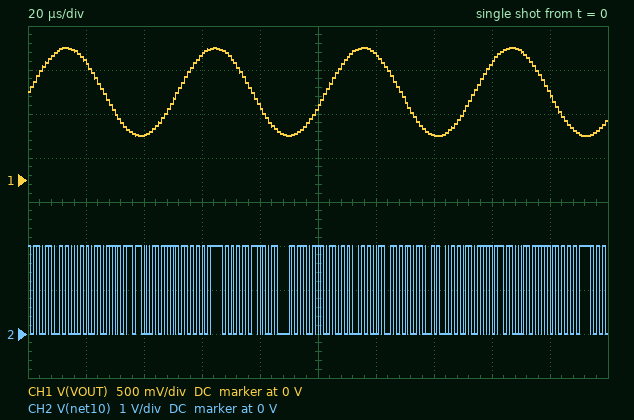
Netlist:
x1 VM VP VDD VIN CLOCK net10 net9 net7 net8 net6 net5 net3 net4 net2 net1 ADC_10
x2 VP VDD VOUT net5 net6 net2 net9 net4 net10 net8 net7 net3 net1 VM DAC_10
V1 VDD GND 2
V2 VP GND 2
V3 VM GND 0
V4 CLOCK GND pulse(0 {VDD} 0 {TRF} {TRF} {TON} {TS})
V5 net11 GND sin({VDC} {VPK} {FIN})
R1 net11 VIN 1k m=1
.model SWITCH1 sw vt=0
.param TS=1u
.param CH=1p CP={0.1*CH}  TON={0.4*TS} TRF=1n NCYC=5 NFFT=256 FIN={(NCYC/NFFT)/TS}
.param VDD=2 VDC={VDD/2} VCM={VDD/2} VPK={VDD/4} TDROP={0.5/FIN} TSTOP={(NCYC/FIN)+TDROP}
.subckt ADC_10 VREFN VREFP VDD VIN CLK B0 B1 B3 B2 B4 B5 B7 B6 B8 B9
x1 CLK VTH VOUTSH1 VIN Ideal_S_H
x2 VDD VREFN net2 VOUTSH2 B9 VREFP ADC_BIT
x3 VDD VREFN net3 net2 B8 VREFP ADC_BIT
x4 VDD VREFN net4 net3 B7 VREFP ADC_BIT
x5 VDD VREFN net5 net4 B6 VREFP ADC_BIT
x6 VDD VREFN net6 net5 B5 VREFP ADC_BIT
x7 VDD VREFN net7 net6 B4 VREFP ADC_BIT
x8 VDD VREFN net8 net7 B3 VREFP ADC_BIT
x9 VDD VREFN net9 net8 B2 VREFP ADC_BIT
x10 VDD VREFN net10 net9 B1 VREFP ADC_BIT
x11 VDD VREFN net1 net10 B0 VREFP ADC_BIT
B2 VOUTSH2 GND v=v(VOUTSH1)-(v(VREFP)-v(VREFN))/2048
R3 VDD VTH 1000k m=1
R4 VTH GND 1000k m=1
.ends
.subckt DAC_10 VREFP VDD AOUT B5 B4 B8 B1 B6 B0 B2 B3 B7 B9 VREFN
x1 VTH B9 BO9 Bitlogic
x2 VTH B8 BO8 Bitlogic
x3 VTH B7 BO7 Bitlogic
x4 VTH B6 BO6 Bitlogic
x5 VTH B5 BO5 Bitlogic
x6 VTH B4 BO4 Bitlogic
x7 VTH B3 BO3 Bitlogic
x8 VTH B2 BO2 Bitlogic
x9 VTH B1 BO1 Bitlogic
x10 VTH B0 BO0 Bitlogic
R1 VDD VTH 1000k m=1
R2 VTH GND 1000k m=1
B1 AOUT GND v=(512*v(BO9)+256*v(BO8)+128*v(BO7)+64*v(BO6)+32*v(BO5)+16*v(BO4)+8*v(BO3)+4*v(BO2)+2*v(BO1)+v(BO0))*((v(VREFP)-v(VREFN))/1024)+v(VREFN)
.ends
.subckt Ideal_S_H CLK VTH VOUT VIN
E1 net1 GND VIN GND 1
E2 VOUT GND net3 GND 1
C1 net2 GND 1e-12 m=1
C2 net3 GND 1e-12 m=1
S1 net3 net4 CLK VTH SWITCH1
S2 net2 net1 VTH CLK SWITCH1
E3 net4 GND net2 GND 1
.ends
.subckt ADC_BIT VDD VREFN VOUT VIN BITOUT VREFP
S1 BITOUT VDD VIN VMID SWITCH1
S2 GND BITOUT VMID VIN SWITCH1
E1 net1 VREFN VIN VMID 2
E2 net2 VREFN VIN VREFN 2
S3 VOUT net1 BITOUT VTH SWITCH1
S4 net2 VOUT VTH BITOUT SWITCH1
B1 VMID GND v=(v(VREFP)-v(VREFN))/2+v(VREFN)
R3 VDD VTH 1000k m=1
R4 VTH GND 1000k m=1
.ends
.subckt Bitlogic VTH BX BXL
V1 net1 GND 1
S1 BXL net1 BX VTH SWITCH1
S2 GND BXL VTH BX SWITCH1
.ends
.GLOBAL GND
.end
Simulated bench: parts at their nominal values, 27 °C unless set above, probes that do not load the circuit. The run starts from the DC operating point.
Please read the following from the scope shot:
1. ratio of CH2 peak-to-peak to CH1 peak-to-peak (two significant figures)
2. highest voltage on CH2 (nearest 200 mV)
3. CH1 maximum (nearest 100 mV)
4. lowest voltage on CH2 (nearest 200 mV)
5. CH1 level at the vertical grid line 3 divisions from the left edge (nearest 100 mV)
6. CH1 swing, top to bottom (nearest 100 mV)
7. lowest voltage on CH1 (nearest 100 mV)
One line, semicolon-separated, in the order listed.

2.0; 2.0 V; 1.5 V; 0 V; 1.4 V; 1.0 V; 500 mV
